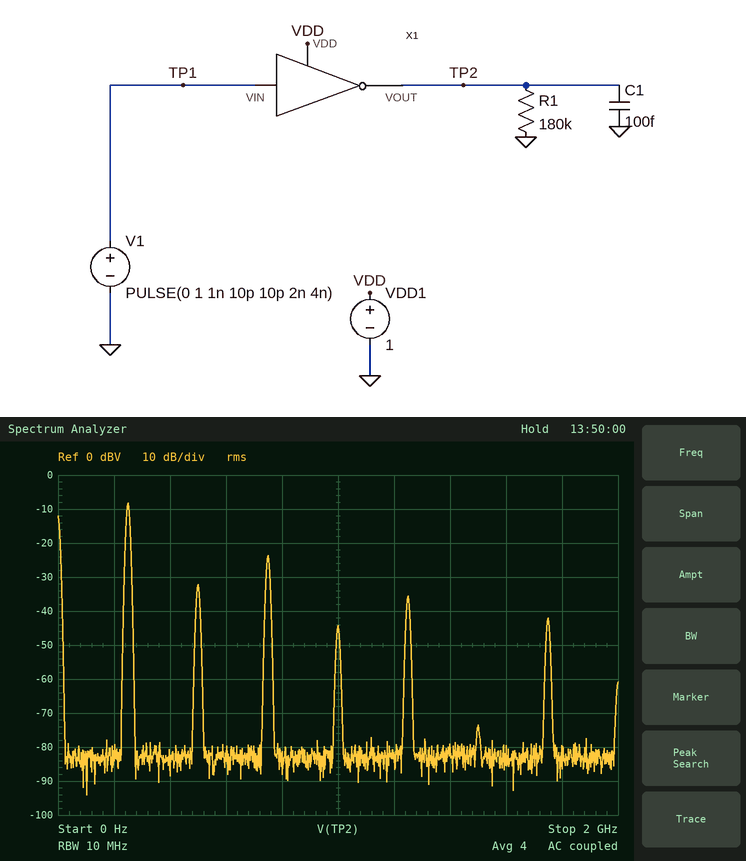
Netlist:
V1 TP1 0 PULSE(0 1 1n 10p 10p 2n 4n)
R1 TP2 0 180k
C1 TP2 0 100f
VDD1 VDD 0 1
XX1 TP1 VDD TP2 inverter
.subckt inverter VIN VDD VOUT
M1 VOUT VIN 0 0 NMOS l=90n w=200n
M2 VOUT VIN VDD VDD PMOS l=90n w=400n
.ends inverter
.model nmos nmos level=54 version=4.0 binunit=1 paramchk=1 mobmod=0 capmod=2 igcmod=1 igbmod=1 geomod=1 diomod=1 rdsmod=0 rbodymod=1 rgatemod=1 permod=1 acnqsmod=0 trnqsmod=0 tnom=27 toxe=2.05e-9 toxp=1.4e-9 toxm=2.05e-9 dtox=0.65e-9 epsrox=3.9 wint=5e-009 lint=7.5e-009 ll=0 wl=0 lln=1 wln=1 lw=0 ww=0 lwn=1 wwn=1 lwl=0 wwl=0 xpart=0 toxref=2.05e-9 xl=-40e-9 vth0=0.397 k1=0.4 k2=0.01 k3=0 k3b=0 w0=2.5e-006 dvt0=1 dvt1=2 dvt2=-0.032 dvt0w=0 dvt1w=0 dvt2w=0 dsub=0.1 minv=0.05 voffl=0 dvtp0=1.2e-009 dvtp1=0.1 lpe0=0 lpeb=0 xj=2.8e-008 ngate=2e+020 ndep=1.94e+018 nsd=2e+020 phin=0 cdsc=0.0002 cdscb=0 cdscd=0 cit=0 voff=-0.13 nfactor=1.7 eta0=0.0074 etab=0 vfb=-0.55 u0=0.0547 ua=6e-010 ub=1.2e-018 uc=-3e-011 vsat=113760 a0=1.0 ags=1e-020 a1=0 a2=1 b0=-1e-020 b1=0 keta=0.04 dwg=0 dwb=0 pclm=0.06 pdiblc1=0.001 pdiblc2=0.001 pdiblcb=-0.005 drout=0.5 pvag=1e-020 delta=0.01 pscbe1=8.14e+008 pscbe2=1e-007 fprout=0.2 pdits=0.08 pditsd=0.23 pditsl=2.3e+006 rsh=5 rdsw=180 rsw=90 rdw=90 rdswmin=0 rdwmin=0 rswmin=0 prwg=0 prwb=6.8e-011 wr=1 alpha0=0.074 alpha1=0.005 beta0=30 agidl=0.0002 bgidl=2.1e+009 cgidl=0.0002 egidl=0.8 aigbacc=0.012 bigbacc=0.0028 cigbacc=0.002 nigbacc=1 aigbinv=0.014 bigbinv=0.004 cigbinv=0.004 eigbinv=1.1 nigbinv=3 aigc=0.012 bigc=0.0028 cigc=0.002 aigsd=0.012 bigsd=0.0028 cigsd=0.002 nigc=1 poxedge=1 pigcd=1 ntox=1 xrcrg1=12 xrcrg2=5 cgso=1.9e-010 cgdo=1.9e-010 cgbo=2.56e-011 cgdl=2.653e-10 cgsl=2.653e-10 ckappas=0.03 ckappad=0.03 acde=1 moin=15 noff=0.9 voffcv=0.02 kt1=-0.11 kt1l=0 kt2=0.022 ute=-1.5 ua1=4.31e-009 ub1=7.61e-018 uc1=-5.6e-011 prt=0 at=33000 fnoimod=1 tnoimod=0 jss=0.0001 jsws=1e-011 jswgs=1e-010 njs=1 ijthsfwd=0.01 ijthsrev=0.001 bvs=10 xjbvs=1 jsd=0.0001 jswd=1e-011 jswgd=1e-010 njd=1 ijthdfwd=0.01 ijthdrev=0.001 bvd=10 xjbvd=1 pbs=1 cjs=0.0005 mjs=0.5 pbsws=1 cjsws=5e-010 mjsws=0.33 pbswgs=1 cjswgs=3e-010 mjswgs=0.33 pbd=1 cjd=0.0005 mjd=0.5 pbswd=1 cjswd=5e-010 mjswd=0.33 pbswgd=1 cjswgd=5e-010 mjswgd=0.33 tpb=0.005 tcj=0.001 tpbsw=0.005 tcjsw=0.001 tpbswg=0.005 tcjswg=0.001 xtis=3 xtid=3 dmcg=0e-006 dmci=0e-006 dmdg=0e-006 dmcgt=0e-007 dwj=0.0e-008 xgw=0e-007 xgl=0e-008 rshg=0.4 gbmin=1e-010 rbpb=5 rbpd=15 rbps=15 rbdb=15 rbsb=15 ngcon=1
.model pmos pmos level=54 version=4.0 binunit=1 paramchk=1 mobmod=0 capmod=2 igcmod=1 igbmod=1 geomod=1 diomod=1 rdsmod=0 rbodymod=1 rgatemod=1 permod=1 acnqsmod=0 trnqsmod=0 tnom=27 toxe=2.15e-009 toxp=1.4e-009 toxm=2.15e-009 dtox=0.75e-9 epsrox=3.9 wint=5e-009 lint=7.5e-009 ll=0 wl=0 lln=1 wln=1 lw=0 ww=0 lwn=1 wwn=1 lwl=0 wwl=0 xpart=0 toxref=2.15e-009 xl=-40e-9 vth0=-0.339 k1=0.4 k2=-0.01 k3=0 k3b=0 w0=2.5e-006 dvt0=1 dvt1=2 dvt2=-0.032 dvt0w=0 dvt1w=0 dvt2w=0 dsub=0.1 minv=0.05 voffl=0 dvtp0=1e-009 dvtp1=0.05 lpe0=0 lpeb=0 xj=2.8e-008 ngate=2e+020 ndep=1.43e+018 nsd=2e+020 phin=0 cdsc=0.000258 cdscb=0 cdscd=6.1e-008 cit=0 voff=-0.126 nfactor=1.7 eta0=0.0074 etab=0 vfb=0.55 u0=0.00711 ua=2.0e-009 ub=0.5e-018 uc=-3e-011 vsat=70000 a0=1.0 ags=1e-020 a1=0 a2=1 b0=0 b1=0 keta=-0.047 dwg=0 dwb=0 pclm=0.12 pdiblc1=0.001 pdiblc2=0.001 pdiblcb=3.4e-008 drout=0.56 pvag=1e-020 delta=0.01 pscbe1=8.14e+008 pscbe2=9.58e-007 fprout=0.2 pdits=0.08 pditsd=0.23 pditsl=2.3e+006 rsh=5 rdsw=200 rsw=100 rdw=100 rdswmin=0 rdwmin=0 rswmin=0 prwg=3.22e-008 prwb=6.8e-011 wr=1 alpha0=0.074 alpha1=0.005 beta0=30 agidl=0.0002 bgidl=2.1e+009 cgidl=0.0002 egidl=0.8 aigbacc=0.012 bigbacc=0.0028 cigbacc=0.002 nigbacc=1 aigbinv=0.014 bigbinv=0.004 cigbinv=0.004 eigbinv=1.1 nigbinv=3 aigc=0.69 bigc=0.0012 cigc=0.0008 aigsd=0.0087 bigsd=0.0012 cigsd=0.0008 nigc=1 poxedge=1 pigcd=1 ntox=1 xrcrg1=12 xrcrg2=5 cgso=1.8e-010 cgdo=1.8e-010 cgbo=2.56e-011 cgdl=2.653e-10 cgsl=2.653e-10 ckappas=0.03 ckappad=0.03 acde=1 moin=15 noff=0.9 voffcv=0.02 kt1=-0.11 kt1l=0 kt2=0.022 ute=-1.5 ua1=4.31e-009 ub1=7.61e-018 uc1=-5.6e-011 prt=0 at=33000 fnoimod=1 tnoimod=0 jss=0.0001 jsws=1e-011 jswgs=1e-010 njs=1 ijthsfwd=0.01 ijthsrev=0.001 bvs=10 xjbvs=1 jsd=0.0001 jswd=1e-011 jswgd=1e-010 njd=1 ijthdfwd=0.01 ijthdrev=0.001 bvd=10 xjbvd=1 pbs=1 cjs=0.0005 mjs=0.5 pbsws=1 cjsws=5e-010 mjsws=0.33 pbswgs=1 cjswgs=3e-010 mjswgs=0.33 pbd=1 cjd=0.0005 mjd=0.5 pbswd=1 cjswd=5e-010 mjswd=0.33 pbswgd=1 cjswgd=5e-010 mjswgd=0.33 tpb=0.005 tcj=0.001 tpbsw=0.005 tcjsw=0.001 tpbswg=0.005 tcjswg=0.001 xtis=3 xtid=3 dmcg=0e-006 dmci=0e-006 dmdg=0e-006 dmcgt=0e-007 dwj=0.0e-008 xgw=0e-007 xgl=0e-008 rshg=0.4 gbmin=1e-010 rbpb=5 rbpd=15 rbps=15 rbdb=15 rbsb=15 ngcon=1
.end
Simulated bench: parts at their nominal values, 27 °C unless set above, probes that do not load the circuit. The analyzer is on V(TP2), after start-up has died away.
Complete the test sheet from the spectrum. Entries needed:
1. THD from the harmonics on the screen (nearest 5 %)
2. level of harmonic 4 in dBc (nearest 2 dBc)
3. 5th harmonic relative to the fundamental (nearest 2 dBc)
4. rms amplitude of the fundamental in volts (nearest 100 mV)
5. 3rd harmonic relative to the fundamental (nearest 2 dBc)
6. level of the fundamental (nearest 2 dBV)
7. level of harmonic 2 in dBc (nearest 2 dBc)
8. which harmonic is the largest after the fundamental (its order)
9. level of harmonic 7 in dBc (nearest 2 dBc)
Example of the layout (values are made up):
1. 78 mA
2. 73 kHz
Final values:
1. 20 %
2. -36 dBc
3. -28 dBc
4. 400 mV
5. -16 dBc
6. -8 dBV
7. -24 dBc
8. 3
9. -34 dBc
